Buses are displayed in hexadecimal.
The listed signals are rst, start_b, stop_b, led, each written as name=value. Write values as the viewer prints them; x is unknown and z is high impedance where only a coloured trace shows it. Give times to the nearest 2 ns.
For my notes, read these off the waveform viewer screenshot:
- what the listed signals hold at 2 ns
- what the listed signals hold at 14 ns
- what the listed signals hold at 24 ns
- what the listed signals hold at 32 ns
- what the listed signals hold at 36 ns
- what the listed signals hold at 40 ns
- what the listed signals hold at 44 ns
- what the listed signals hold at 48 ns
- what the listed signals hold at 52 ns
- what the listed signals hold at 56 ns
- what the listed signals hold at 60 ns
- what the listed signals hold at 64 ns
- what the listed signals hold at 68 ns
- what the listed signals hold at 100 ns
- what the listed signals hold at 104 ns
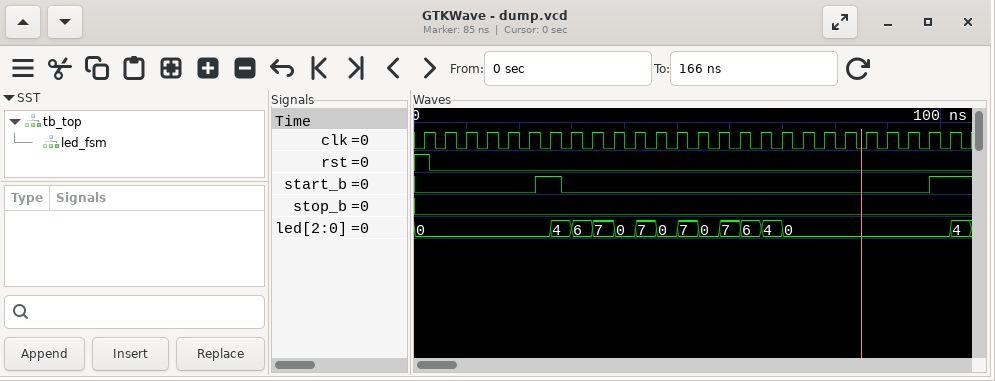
rst=1, start_b=0, stop_b=0, led=0
rst=0, start_b=0, stop_b=0, led=0
rst=0, start_b=1, stop_b=0, led=0
rst=0, start_b=0, stop_b=0, led=6
rst=0, start_b=0, stop_b=0, led=7
rst=0, start_b=0, stop_b=0, led=0
rst=0, start_b=0, stop_b=0, led=7
rst=0, start_b=0, stop_b=0, led=0
rst=0, start_b=0, stop_b=0, led=7
rst=0, start_b=0, stop_b=0, led=0
rst=0, start_b=0, stop_b=0, led=7
rst=0, start_b=0, stop_b=0, led=6
rst=0, start_b=0, stop_b=0, led=4
rst=0, start_b=1, stop_b=0, led=0
rst=0, start_b=1, stop_b=0, led=4
